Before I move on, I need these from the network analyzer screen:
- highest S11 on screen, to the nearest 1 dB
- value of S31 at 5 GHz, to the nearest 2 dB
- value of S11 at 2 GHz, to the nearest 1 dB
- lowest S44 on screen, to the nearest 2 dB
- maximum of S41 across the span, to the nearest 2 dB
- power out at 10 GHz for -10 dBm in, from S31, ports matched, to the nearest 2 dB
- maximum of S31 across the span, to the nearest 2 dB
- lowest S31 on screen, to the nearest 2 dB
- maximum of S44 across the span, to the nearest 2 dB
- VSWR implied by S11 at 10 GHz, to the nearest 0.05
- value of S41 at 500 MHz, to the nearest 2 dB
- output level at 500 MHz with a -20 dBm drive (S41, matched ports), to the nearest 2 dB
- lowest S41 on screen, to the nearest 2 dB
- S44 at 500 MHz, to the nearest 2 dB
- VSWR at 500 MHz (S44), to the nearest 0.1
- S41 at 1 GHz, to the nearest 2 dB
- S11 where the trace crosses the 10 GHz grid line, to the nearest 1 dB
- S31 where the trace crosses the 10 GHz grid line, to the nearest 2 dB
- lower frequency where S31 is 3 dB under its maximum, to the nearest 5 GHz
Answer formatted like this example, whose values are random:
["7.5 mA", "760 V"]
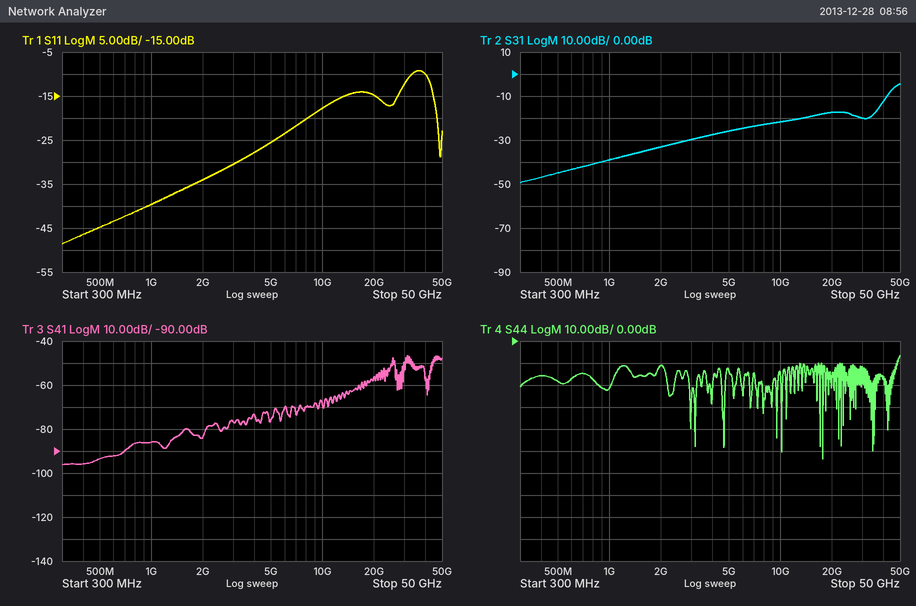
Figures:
["-9 dB", "-26 dB", "-34 dB", "-54 dB", "-46 dB", "-32 dBm", "-4 dB", "-50 dB", "-6 dB", "1.30", "-94 dB", "-114 dBm", "-96 dB", "-18 dB", "1.3", "-86 dB", "-18 dB", "-22 dB", "45 GHz"]
